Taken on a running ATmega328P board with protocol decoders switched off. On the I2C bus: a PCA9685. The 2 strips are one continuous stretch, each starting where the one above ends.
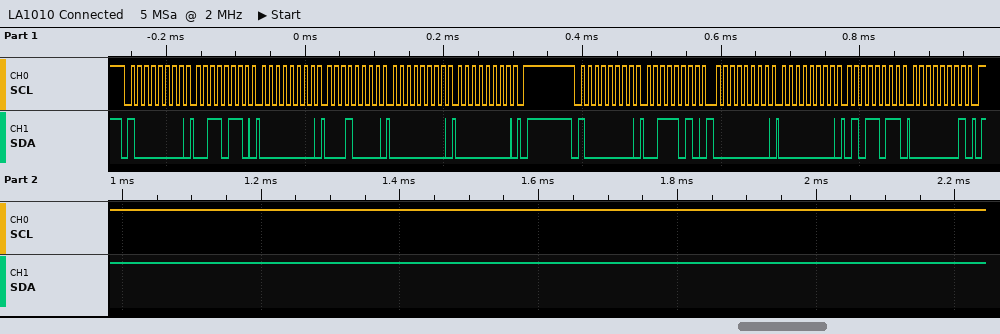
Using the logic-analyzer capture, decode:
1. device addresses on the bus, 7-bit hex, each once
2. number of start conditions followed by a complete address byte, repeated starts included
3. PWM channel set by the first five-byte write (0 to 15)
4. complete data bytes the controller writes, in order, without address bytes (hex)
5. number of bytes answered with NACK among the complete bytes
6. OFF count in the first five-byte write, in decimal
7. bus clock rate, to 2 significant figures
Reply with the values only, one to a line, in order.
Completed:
0x40
2
12
36 00 10 00 00 3A 00 00 5B 01
0
0
100 kHz
